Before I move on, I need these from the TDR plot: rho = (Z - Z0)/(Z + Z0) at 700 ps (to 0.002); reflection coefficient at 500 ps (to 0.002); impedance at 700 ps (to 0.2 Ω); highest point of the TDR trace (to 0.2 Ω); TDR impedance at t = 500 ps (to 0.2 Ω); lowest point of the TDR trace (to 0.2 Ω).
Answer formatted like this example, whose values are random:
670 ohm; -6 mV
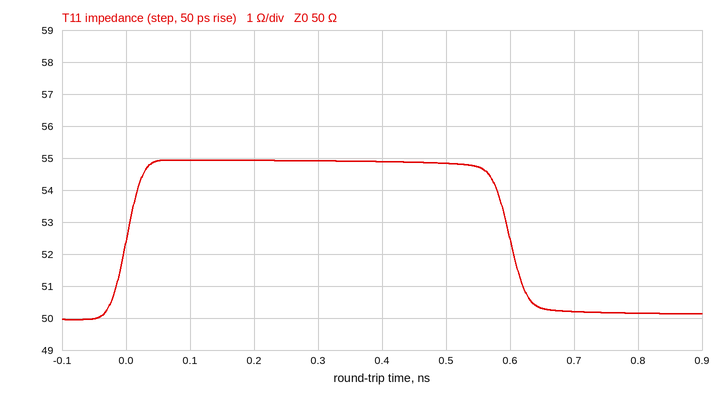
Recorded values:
+0.002; +0.046; 50.2 Ω; 55.0 Ω; 54.8 Ω; 50.0 Ω
